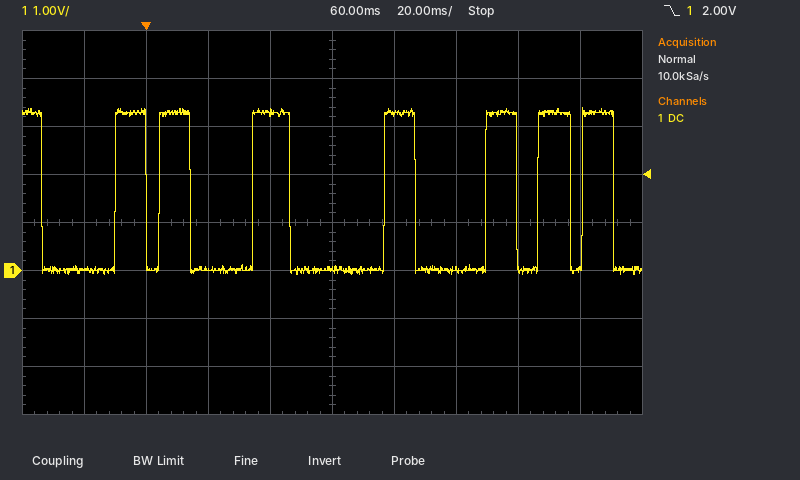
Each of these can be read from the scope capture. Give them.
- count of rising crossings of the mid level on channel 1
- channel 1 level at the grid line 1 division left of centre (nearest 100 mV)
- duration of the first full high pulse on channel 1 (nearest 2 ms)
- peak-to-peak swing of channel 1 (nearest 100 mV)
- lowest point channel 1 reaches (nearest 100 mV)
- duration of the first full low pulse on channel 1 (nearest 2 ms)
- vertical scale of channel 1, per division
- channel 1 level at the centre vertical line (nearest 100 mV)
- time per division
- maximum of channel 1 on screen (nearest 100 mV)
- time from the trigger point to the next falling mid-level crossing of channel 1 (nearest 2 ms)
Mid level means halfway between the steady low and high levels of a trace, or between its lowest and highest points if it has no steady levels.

7
3.3 V
10 ms
3.5 V
-100 mV
24 ms
1 V
0.0 V
20 ms
3.4 V
14 ms
